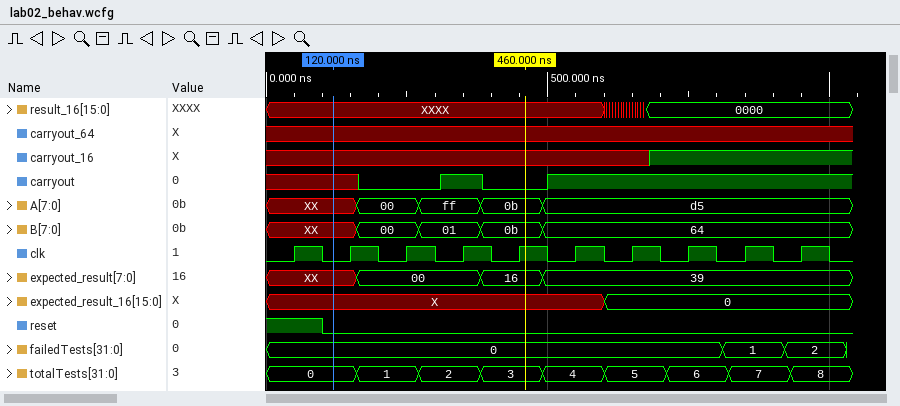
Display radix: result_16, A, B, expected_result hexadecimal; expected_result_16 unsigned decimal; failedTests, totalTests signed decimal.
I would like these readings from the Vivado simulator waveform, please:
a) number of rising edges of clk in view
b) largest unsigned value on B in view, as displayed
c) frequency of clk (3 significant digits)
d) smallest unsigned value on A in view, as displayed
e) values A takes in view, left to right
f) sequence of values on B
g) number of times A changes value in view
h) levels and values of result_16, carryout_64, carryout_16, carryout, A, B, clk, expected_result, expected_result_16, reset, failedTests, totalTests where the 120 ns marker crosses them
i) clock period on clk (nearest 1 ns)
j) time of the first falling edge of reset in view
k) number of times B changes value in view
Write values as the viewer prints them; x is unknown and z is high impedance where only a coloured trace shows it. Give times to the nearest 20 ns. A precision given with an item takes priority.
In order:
10
64
10.0 MHz
00
XX, 00, ff, 0b, d5
XX, 00, 01, 0b, 64
4
result_16=XXXX, carryout_64=x, carryout_16=x, carryout=x, A=XX, B=XX, clk=0, expected_result=XX, expected_result_16=X, reset=0, failedTests=0, totalTests=0
100 ns
100 ns
4
